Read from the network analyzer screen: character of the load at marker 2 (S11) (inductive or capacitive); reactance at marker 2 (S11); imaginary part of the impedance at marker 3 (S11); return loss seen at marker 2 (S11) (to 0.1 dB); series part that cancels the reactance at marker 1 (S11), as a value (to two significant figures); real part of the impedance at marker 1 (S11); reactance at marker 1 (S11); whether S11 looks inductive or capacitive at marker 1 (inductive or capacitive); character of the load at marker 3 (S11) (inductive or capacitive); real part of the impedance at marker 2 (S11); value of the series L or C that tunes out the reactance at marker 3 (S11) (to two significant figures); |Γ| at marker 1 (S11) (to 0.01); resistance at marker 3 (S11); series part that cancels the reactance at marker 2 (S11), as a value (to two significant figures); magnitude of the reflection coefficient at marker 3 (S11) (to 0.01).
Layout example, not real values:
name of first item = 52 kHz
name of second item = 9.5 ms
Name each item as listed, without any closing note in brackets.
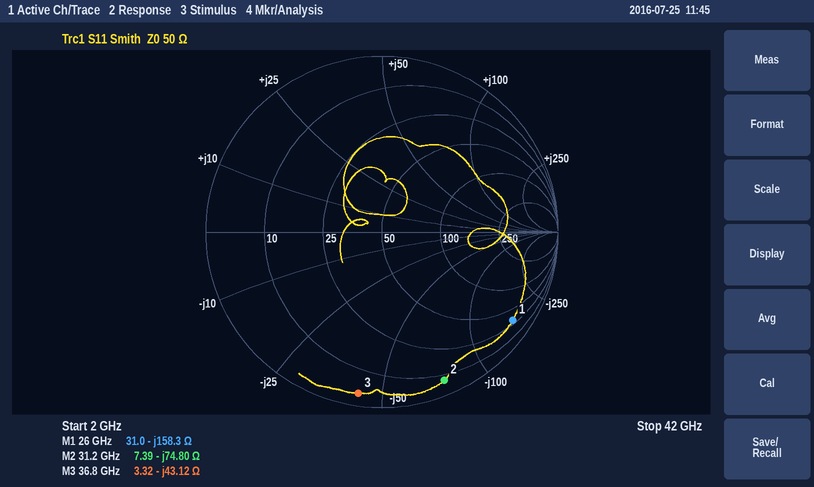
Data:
character of the load at marker 2 (S11) = capacitive
reactance at marker 2 = -74.80 Ω
imaginary part of the impedance at marker 3 = -43.12 Ω
return loss seen at marker 2 (S11) = 0.8 dB
series part that cancels the reactance at marker 1 (S11), as a value = 970 pH
real part of the impedance at marker 1 = 31.0 Ω
reactance at marker 1 = -158.3 Ω
whether S11 looks inductive or capacitive at marker 1 = capacitive
character of the load at marker 3 (S11) = capacitive
real part of the impedance at marker 2 = 7.39 Ω
value of the series L or C that tunes out the reactance at marker 3 (S11) = 190 pH
|Γ| at marker 1 (S11) = 0.90
resistance at marker 3 = 3.32 Ω
series part that cancels the reactance at marker 2 (S11), as a value = 380 pH
magnitude of the reflection coefficient at marker 3 (S11) = 0.93
